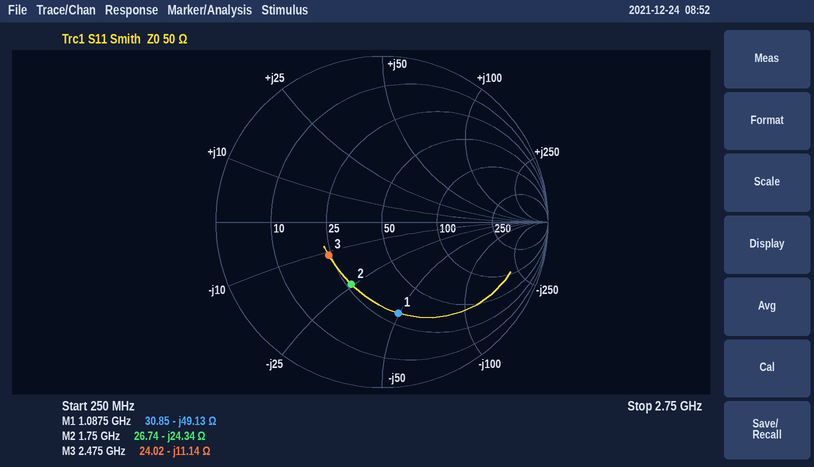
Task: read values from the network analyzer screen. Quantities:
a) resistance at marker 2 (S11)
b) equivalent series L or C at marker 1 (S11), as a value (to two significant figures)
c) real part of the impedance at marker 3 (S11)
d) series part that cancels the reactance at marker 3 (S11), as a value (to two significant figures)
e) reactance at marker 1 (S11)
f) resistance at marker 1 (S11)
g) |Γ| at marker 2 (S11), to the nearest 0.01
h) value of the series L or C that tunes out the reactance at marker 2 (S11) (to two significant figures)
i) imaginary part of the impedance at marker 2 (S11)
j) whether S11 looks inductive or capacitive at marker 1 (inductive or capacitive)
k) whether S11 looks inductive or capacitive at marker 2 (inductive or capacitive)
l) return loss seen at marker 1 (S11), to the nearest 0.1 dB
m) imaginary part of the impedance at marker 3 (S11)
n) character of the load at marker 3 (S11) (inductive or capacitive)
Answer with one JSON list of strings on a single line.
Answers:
["26.74 Ω", "3.0 pF", "24.02 Ω", "720 pH", "-49.13 Ω", "30.85 Ω", "0.42", "2.2 nH", "-24.34 Ω", "capacitive", "capacitive", "5.1 dB", "-11.14 Ω", "capacitive"]
